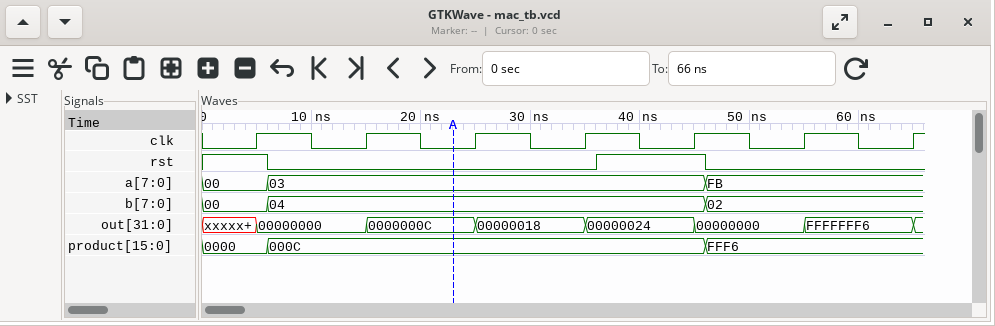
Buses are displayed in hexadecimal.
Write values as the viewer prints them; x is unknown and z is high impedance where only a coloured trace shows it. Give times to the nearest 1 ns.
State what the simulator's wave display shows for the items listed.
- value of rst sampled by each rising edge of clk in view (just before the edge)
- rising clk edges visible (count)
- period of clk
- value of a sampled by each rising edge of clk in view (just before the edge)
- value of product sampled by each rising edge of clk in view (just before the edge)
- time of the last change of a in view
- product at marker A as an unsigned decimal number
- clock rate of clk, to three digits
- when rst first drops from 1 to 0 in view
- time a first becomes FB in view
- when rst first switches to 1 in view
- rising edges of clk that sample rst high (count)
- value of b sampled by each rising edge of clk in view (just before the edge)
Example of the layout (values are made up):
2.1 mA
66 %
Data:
1 0 0 0 1 0 0
7
10 ns
00, 03, 03, 03, 03, FB, FB
0000, 000C, 000C, 000C, 000C, FFF6, FFF6
46 ns
12
100 MHz
6 ns
46 ns
36 ns
2
00, 04, 04, 04, 04, 02, 02
